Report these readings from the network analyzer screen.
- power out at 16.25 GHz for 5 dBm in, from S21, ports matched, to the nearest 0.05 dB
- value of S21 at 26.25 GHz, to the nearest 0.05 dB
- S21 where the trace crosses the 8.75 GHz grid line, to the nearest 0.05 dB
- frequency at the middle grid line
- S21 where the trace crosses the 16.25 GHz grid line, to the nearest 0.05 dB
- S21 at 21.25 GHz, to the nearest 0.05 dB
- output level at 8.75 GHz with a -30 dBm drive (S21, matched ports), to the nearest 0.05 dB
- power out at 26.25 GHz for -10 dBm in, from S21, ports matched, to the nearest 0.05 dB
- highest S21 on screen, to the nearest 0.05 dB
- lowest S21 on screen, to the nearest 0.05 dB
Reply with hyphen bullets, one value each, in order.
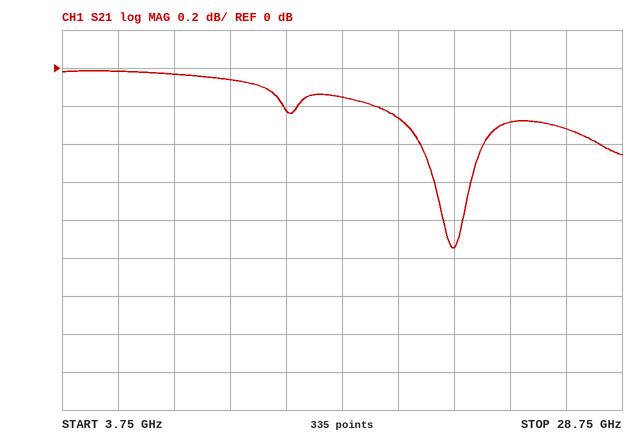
- 4.85 dBm
- -0.30 dB
- -0.05 dB
- 16.25 GHz
- -0.15 dB
- -0.95 dB
- -30.05 dBm
- -10.30 dBm
- 0.00 dB
- -0.95 dB
